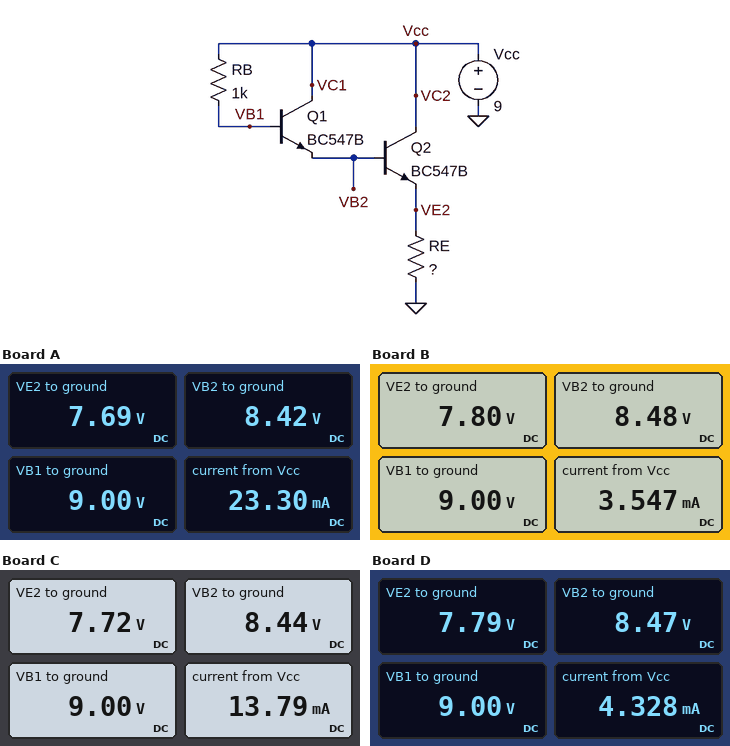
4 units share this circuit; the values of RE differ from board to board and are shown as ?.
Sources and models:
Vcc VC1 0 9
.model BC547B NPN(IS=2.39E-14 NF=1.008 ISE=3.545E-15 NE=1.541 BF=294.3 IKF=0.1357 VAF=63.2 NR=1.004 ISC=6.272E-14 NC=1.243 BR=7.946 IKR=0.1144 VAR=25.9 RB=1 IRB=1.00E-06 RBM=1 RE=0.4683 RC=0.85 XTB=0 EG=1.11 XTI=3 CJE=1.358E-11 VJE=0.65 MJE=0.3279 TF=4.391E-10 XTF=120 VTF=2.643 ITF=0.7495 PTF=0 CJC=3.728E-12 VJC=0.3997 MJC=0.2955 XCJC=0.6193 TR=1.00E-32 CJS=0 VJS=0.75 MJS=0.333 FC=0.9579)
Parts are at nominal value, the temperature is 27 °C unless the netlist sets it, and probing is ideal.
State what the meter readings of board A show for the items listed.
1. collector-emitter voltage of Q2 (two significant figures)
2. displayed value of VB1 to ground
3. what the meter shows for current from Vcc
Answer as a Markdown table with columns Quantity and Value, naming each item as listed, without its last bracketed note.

| Quantity | Value |
|---|---|
| collector-emitter voltage of Q2 | 1.3 V |
| displayed value of VB1 to ground | 9.00 V |
| what the meter shows for current from Vcc | 23.30 mA |
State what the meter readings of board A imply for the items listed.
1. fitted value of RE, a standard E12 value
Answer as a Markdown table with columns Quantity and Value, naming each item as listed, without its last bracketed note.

| Quantity | Value |
|---|---|
| fitted value of RE, a standard E12 value | 330 Ω |
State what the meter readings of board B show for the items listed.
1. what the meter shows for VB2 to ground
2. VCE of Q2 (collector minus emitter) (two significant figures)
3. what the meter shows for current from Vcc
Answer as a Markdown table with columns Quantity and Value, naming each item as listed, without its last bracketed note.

| Quantity | Value |
|---|---|
| what the meter shows for VB2 to ground | 8.48 V |
| VCE of Q2 (collector minus emitter) | 1.2 V |
| what the meter shows for current from Vcc | 3.547 mA |
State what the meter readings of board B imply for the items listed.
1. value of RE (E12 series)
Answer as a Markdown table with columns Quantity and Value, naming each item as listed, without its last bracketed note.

| Quantity | Value |
|---|---|
| value of RE | 2.2 kΩ |
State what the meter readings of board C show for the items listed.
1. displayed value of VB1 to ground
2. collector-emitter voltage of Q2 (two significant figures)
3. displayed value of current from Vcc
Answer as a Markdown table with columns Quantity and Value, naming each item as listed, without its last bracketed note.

| Quantity | Value |
|---|---|
| displayed value of VB1 to ground | 9.00 V |
| collector-emitter voltage of Q2 | 1.3 V |
| displayed value of current from Vcc | 13.79 mA |
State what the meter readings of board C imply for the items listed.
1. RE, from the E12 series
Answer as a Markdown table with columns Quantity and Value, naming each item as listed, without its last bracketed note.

| Quantity | Value |
|---|---|
| RE, from the E12 series | 560 Ω |
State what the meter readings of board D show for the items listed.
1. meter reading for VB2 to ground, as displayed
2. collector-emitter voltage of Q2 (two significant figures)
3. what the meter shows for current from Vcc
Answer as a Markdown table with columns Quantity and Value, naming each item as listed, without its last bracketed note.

| Quantity | Value |
|---|---|
| meter reading for VB2 to ground, as displayed | 8.47 V |
| collector-emitter voltage of Q2 | 1.2 V |
| what the meter shows for current from Vcc | 4.328 mA |
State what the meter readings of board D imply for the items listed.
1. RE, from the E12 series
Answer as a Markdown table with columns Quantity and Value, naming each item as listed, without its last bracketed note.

| Quantity | Value |
|---|---|
| RE, from the E12 series | 1.8 kΩ |
